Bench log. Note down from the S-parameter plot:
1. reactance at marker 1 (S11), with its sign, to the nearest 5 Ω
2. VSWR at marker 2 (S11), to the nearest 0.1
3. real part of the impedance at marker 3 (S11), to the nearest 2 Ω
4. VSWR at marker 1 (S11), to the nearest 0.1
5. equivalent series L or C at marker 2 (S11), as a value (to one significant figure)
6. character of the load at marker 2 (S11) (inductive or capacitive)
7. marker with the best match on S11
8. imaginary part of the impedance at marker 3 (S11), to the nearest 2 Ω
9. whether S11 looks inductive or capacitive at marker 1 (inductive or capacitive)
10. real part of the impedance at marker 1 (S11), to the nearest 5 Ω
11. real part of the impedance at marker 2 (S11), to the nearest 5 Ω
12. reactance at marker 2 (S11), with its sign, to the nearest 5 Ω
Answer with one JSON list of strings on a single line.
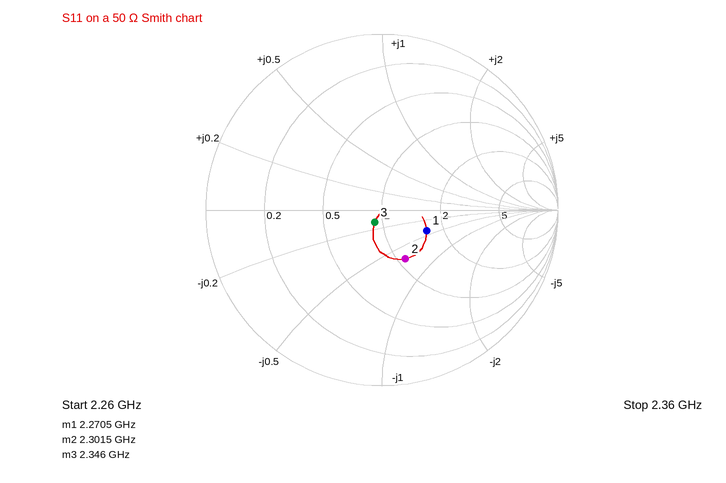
["-20 Ω", "1.9", "46 Ω", "1.8", "2 pF", "capacitive", "marker 3", "-6 Ω", "capacitive", "80 Ω", "55 Ω", "-35 Ω"]
